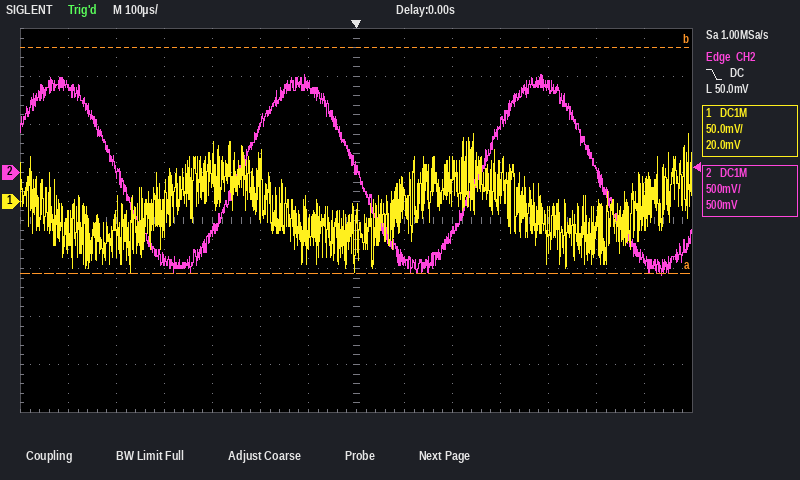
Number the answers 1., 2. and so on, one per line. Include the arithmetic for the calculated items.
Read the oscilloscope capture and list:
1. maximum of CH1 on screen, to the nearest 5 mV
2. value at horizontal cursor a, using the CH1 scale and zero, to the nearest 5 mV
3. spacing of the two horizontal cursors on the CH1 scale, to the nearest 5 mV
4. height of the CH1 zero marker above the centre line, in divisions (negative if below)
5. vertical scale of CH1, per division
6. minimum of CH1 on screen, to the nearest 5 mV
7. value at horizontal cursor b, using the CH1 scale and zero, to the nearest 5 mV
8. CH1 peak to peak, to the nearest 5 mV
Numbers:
1. 70 mV
2. -75 mV
3. 235 mV
4. +0.4 div
5. 50 mV
6. -75 mV
7. 160 mV
8. 70 mV − (-75 mV) = 145 mV
